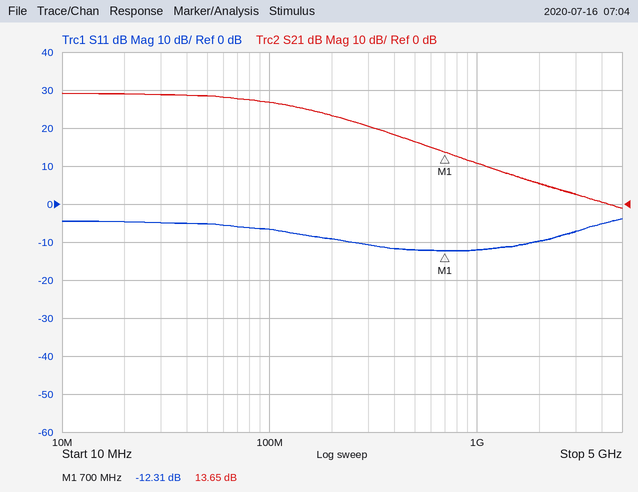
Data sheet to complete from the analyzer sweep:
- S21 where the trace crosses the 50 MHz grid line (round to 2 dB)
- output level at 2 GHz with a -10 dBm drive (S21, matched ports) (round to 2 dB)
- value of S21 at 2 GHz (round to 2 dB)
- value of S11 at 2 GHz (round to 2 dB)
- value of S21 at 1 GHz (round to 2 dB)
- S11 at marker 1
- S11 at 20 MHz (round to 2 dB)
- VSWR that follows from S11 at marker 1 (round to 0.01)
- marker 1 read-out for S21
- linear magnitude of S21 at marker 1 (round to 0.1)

28 dB
-4 dBm
6 dB
-10 dB
10 dB
-12.31 dB
-4 dB
1.64
13.65 dB
4.8
